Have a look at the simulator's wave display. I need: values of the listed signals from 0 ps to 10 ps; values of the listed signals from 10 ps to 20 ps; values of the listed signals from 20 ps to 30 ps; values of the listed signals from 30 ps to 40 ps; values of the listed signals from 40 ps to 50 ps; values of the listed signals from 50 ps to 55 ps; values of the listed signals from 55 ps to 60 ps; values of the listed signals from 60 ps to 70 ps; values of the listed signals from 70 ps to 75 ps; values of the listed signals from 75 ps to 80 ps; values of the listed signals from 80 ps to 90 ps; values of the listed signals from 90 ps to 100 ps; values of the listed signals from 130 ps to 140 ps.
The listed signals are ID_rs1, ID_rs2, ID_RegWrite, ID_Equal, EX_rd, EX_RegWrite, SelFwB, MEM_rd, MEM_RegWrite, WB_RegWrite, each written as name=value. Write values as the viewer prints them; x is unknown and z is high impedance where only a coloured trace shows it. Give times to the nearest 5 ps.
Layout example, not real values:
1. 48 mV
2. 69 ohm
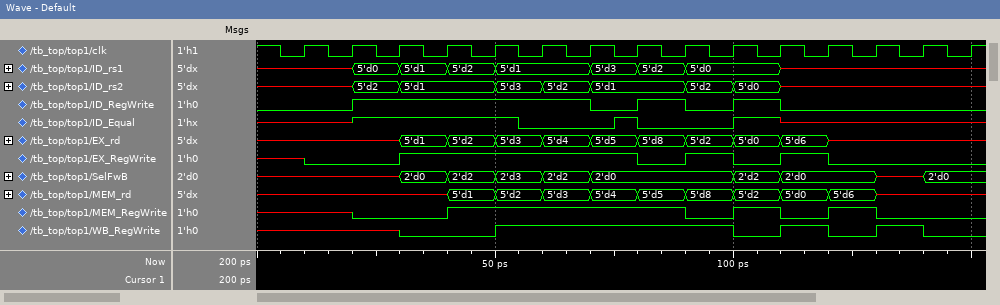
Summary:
1. ID_rs1=x, ID_rs2=x, ID_RegWrite=0, ID_Equal=x, EX_rd=x, EX_RegWrite=x, SelFwB=x, MEM_rd=x, MEM_RegWrite=x, WB_RegWrite=x
2. ID_rs1=x, ID_rs2=x, ID_RegWrite=0, ID_Equal=x, EX_rd=x, EX_RegWrite=0, SelFwB=x, MEM_rd=x, MEM_RegWrite=x, WB_RegWrite=x
3. ID_rs1=5'd0, ID_rs2=5'd2, ID_RegWrite=1, ID_Equal=1, EX_rd=x, EX_RegWrite=0, SelFwB=x, MEM_rd=x, MEM_RegWrite=0, WB_RegWrite=x
4. ID_rs1=5'd1, ID_rs2=5'd1, ID_RegWrite=1, ID_Equal=1, EX_rd=5'd1, EX_RegWrite=1, SelFwB=2'd0, MEM_rd=x, MEM_RegWrite=0, WB_RegWrite=0
5. ID_rs1=5'd2, ID_rs2=5'd1, ID_RegWrite=1, ID_Equal=1, EX_rd=5'd2, EX_RegWrite=1, SelFwB=2'd2, MEM_rd=5'd1, MEM_RegWrite=1, WB_RegWrite=0
6. ID_rs1=5'd1, ID_rs2=5'd3, ID_RegWrite=1, ID_Equal=1, EX_rd=5'd3, EX_RegWrite=1, SelFwB=2'd3, MEM_rd=5'd2, MEM_RegWrite=1, WB_RegWrite=1
7. ID_rs1=5'd1, ID_rs2=5'd3, ID_RegWrite=1, ID_Equal=0, EX_rd=5'd3, EX_RegWrite=1, SelFwB=2'd3, MEM_rd=5'd2, MEM_RegWrite=1, WB_RegWrite=1
8. ID_rs1=5'd1, ID_rs2=5'd2, ID_RegWrite=1, ID_Equal=0, EX_rd=5'd4, EX_RegWrite=1, SelFwB=2'd2, MEM_rd=5'd3, MEM_RegWrite=1, WB_RegWrite=1
9. ID_rs1=5'd3, ID_rs2=5'd1, ID_RegWrite=0, ID_Equal=0, EX_rd=5'd5, EX_RegWrite=1, SelFwB=2'd0, MEM_rd=5'd4, MEM_RegWrite=1, WB_RegWrite=1
10. ID_rs1=5'd3, ID_rs2=5'd1, ID_RegWrite=0, ID_Equal=1, EX_rd=5'd5, EX_RegWrite=1, SelFwB=2'd0, MEM_rd=5'd4, MEM_RegWrite=1, WB_RegWrite=1
11. ID_rs1=5'd2, ID_rs2=5'd1, ID_RegWrite=1, ID_Equal=0, EX_rd=5'd8, EX_RegWrite=0, SelFwB=2'd0, MEM_rd=5'd5, MEM_RegWrite=1, WB_RegWrite=1
12. ID_rs1=5'd0, ID_rs2=5'd2, ID_RegWrite=0, ID_Equal=0, EX_rd=5'd2, EX_RegWrite=1, SelFwB=2'd0, MEM_rd=5'd8, MEM_RegWrite=0, WB_RegWrite=1
13. ID_rs1=x, ID_rs2=x, ID_RegWrite=0, ID_Equal=x, EX_rd=x, EX_RegWrite=0, SelFwB=x, MEM_rd=x, MEM_RegWrite=0, WB_RegWrite=1
